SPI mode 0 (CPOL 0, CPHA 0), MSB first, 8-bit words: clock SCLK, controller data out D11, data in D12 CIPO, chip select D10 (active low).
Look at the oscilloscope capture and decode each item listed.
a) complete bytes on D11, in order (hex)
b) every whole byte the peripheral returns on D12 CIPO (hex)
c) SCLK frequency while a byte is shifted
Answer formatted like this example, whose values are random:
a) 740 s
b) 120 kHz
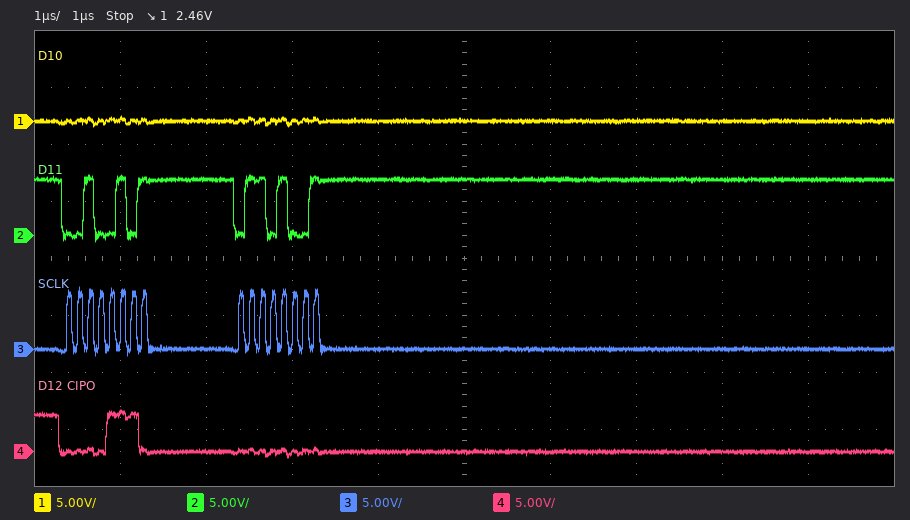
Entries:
a) 25 69
b) 0E 00
c) 8 MHz
